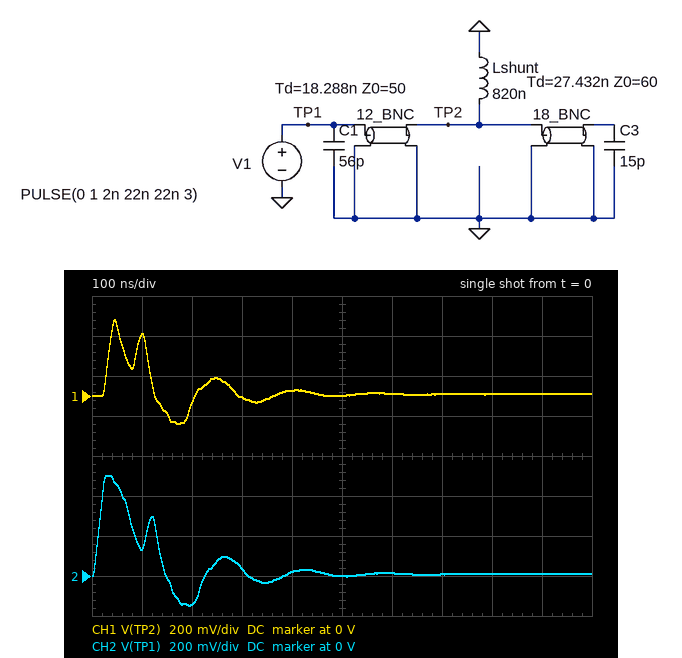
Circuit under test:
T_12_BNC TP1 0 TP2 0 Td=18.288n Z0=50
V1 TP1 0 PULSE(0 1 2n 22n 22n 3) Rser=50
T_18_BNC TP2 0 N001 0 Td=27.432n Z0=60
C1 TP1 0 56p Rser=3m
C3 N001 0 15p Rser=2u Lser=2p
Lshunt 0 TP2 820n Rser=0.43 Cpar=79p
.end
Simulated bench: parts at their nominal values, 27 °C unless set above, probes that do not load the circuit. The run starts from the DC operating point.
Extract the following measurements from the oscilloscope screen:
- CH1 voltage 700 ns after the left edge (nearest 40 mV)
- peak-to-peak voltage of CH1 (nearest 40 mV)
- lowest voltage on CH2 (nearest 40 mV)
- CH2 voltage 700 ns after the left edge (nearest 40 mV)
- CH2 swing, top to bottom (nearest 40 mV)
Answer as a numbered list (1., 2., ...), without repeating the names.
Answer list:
1. 0 V
2. 520 mV
3. -160 mV
4. 0 V
5. 640 mV
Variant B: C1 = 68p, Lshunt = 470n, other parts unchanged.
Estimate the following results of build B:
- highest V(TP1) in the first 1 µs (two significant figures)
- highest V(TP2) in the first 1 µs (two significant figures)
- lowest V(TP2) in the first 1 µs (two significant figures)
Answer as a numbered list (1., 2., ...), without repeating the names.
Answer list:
1. 500 mV
2. 310 mV
3. -110 mV
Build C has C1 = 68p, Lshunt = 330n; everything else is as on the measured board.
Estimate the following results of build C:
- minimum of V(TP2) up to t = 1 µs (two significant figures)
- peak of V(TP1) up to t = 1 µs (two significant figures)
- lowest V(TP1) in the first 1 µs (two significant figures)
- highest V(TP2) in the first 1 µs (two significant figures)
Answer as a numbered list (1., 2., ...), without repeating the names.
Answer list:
1. -88 mV
2. 500 mV
3. -84 mV
4. 260 mV
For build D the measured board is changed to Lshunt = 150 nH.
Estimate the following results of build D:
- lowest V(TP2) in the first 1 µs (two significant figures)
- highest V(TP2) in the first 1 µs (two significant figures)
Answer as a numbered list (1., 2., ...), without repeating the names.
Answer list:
1. -45 mV
2. 140 mV
